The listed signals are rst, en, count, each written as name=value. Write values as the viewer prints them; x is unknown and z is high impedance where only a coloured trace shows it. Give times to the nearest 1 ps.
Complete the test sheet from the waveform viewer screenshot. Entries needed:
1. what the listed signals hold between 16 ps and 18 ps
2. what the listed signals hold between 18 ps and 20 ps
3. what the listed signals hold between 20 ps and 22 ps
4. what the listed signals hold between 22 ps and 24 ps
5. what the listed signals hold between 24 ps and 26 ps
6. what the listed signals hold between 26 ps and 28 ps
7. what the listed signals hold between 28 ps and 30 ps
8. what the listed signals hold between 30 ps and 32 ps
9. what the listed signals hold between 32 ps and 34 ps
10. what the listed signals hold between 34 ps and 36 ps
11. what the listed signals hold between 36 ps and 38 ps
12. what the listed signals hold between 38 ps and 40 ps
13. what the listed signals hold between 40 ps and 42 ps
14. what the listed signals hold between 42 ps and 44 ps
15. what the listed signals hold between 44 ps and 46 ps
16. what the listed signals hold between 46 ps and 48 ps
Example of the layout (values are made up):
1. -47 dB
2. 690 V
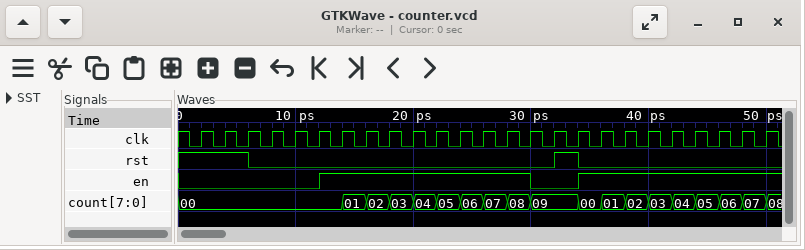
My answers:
1. rst=0, en=1, count=02
2. rst=0, en=1, count=03
3. rst=0, en=1, count=04
4. rst=0, en=1, count=05
5. rst=0, en=1, count=06
6. rst=0, en=1, count=07
7. rst=0, en=1, count=08
8. rst=0, en=0, count=09
9. rst=1, en=0, count=09
10. rst=0, en=1, count=00
11. rst=0, en=1, count=01
12. rst=0, en=1, count=02
13. rst=0, en=1, count=03
14. rst=0, en=1, count=04
15. rst=0, en=1, count=05
16. rst=0, en=1, count=06
